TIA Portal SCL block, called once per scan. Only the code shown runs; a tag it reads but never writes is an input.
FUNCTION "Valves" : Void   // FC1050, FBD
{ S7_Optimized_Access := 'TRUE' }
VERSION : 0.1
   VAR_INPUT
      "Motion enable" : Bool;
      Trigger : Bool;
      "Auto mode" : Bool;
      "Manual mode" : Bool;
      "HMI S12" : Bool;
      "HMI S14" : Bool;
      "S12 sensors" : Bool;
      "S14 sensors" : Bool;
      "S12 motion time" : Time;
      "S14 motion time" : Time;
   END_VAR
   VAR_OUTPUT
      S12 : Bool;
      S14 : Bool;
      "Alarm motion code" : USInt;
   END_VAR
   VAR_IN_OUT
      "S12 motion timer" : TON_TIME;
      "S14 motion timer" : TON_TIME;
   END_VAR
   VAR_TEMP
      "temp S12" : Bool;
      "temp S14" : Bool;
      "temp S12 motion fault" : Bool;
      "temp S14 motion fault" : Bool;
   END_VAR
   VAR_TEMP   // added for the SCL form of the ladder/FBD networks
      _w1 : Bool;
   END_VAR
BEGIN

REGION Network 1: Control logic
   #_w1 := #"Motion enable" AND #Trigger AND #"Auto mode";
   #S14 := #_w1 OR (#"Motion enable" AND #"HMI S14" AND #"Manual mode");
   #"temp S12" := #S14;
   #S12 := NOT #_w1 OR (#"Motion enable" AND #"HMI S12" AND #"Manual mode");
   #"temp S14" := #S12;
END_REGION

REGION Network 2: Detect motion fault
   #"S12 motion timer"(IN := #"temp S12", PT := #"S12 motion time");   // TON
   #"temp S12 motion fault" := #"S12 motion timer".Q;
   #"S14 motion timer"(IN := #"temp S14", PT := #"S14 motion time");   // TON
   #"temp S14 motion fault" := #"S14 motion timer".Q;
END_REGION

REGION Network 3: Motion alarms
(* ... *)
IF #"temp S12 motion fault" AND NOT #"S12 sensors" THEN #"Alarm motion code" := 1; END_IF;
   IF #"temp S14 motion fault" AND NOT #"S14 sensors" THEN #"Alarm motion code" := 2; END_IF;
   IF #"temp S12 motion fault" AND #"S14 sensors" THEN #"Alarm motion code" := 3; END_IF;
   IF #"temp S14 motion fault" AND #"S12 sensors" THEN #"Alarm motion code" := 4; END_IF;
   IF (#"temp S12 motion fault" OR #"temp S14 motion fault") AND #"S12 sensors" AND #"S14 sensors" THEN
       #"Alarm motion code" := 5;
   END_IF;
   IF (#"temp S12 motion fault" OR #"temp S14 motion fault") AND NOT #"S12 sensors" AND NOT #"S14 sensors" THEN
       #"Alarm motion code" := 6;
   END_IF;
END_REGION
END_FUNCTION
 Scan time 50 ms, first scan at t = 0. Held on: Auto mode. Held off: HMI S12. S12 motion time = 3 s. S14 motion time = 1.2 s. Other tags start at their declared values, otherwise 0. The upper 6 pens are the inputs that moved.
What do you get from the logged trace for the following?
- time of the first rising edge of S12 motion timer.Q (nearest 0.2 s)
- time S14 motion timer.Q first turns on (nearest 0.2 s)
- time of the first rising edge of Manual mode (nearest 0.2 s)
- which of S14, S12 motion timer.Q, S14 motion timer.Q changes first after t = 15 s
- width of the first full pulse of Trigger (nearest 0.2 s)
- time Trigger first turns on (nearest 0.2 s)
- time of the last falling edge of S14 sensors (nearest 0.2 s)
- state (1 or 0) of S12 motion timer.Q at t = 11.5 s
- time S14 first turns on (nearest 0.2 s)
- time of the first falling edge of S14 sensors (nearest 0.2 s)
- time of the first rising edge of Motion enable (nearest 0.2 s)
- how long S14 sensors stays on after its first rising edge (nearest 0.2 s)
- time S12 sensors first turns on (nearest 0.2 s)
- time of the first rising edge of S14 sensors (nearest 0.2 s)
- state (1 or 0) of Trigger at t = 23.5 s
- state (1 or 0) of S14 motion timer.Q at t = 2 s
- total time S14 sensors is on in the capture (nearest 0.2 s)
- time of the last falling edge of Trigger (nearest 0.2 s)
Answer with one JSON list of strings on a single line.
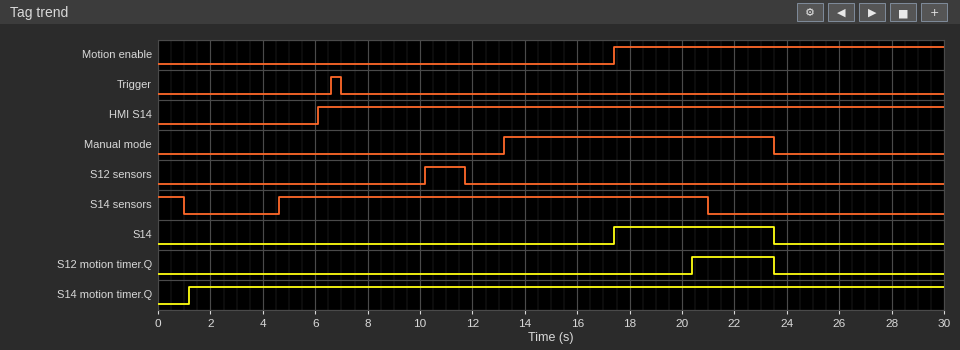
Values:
["20.4 s", "1.2 s", "13.2 s", "S14", "0.4 s", "6.6 s", "21.0 s", "0", "17.4 s", "1.0 s", "17.4 s", "16.4 s", "10.2 s", "4.6 s", "0", "1", "17.4 s", "7.0 s"]
